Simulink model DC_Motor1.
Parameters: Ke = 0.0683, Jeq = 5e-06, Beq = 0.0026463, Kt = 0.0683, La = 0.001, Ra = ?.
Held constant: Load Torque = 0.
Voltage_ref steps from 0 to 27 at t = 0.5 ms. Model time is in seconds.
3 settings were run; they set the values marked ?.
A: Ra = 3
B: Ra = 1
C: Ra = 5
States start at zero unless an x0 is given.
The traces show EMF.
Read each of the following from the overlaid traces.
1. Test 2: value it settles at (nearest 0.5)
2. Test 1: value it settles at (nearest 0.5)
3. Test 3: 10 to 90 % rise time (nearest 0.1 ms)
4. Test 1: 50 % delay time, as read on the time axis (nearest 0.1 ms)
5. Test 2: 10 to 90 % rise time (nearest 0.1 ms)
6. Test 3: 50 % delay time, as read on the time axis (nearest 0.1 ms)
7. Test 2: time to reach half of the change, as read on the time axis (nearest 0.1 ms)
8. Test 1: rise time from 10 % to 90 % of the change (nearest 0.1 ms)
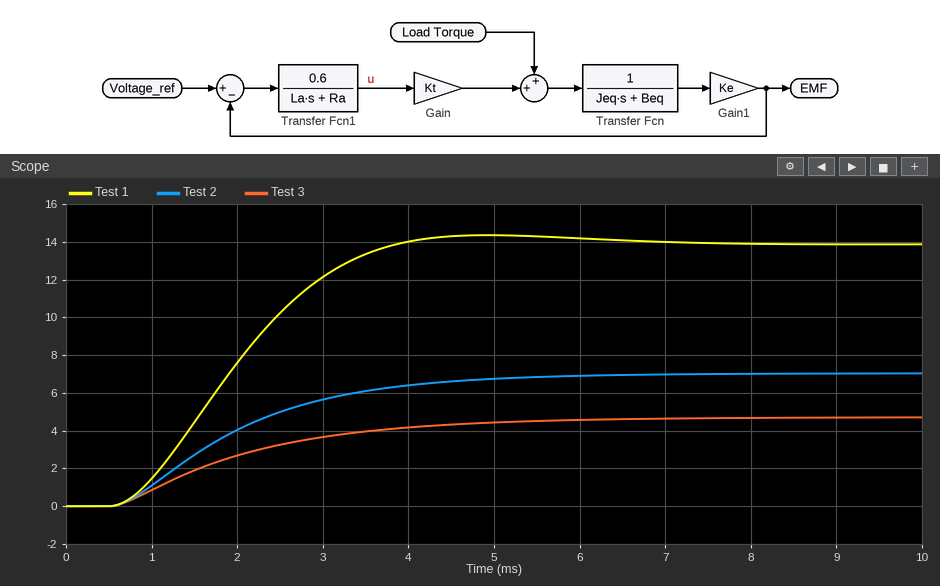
7.0
14.0
3.4 ms
1.9 ms
3.0 ms
1.8 ms
1.8 ms
2.1 ms
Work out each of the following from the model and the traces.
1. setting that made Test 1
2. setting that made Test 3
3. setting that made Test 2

B
C
A
